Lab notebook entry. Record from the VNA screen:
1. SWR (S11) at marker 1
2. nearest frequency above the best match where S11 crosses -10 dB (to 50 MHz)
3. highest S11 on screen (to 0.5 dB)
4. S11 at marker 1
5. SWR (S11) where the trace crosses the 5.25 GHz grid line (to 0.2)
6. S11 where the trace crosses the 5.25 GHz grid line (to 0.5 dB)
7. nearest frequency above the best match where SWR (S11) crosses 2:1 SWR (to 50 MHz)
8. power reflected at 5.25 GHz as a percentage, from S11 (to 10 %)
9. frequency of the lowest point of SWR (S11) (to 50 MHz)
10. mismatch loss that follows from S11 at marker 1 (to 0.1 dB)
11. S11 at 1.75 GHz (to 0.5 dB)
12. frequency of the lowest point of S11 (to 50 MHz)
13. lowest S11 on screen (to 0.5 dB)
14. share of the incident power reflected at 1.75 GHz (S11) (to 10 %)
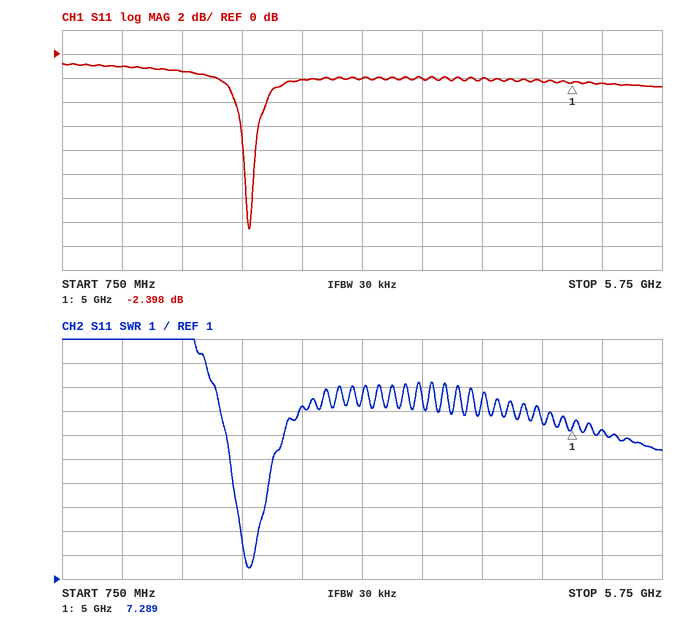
7.289
2.35 GHz
-1.0 dB
-2.398 dB
7.2
-2.5 dB
2.35 GHz
60 %
2.30 GHz
3.7 dB
-1.5 dB
2.30 GHz
-14.5 dB
70 %
